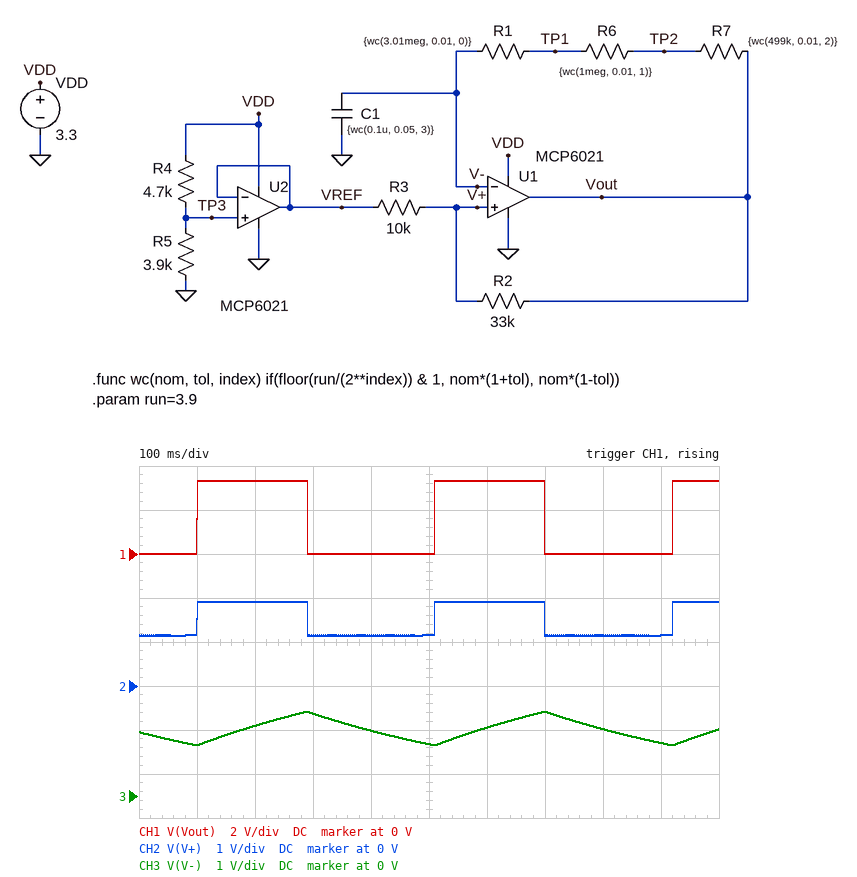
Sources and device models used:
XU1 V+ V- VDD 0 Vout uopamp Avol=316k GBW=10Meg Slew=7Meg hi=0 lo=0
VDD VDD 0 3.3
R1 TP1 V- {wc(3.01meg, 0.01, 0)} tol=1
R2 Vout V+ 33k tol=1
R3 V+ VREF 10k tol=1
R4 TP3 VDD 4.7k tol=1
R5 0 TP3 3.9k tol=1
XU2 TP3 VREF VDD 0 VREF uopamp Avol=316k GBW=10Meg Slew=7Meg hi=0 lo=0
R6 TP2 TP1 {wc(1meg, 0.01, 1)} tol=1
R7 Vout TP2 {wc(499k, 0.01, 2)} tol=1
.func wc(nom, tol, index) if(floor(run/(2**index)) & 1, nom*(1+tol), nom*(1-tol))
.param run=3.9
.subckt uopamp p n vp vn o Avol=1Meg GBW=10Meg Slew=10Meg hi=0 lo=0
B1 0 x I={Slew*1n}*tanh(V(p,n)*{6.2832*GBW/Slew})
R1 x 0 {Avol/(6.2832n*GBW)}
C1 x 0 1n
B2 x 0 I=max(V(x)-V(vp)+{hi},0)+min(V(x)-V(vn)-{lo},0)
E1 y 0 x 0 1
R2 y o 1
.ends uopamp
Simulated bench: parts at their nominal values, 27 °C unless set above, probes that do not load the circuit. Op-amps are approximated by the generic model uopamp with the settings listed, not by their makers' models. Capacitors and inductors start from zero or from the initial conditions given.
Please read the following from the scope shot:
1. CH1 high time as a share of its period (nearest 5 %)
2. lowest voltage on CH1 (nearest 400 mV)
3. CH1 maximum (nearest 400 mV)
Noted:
45 %
0 V
3.2 V
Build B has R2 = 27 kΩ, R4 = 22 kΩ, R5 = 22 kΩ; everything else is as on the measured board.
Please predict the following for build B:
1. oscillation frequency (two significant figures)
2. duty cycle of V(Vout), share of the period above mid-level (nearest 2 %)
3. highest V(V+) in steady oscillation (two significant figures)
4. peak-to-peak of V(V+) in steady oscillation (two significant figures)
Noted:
2.1 Hz
50 %
2.1 V
900 mV
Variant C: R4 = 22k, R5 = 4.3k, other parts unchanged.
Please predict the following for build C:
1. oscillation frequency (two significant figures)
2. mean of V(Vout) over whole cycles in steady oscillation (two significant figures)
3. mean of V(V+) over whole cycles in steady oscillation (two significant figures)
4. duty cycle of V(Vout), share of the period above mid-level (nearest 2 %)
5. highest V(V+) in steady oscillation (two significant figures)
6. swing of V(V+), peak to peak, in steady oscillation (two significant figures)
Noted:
1.7 Hz
750 mV
590 mV
22 %
1.2 V
770 mV
